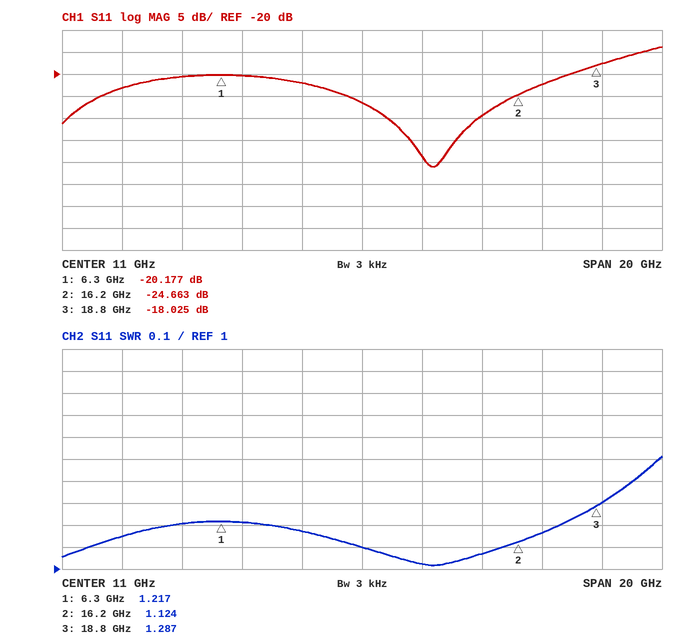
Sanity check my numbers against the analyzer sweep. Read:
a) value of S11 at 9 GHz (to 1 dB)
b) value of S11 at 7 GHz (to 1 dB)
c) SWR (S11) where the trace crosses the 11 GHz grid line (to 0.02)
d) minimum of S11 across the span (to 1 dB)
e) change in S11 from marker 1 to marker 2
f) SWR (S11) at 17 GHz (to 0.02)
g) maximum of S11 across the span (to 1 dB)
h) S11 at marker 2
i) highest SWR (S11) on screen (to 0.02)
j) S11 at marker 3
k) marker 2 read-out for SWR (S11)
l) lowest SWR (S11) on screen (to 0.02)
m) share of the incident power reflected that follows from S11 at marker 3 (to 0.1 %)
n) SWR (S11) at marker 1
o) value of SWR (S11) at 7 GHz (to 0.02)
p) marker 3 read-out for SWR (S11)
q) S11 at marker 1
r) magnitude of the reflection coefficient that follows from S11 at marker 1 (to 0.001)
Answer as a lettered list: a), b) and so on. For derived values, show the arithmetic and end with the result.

a) -22 dB
b) -20 dB
c) 1.10
d) -41 dB
e) -24.663 − (-20.177) = -4.486 dB
f) 1.16
g) -14 dB
h) -24.663 dB
i) 1.52
j) -18.025 dB
k) 1.124
l) 1.02
m) 10^(-18.025/10) ≈ 1.6 %
n) 1.217
o) 1.22
p) 1.287
q) -20.177 dB
r) 10^(-20.177/20) ≈ 0.098
